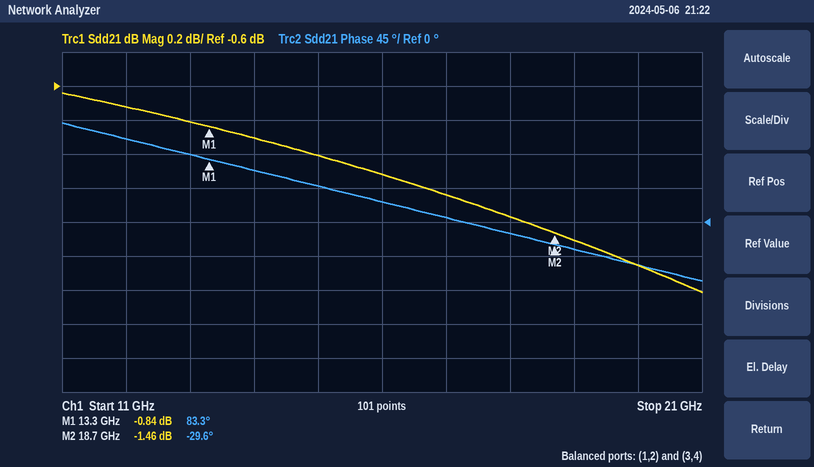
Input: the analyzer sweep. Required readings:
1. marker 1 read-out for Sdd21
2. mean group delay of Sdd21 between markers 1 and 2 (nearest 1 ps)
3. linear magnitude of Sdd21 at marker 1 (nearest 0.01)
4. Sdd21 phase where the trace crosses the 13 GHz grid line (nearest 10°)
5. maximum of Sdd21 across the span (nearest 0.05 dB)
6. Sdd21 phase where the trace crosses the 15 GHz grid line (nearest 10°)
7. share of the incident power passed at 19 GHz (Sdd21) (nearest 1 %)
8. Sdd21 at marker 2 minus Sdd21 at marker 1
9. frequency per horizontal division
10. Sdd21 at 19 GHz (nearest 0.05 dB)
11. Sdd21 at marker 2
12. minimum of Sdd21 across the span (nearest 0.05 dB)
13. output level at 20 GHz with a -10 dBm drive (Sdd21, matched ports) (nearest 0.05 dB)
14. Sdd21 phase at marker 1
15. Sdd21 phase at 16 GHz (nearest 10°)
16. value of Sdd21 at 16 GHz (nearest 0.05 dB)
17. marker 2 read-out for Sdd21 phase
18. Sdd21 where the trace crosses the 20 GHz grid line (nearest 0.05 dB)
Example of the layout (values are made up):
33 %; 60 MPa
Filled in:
-0.84 dB; 58 ps; 0.91; 90°; -0.65 dB; 50°; 71 %; -0.62 dB; 1 GHz; -1.50 dB; -1.46 dB; -1.80 dB; -11.65 dBm; 83.3°; 30°; -1.10 dB; -29.6°; -1.65 dB
